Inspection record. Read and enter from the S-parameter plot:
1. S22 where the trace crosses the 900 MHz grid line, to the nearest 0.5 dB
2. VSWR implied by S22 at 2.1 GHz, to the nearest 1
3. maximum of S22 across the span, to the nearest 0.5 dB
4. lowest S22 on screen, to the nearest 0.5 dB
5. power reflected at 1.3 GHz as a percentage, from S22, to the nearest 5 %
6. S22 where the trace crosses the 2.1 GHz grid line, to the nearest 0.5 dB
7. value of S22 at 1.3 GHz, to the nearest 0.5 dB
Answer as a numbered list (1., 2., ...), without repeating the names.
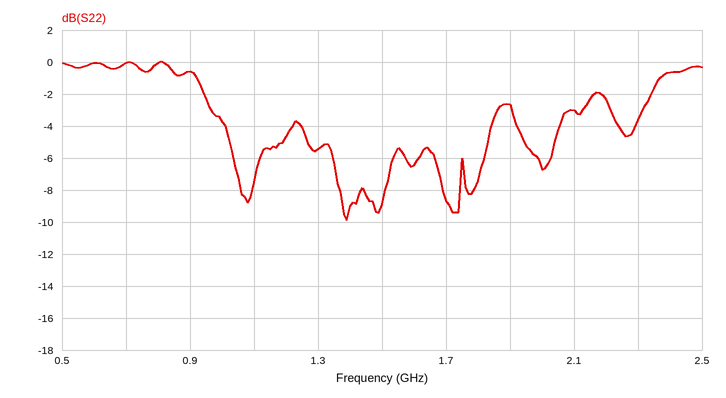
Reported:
1. -0.5 dB
2. 6
3. 0.0 dB
4. -10.0 dB
5. 30 %
6. -3.0 dB
7. -5.5 dB
